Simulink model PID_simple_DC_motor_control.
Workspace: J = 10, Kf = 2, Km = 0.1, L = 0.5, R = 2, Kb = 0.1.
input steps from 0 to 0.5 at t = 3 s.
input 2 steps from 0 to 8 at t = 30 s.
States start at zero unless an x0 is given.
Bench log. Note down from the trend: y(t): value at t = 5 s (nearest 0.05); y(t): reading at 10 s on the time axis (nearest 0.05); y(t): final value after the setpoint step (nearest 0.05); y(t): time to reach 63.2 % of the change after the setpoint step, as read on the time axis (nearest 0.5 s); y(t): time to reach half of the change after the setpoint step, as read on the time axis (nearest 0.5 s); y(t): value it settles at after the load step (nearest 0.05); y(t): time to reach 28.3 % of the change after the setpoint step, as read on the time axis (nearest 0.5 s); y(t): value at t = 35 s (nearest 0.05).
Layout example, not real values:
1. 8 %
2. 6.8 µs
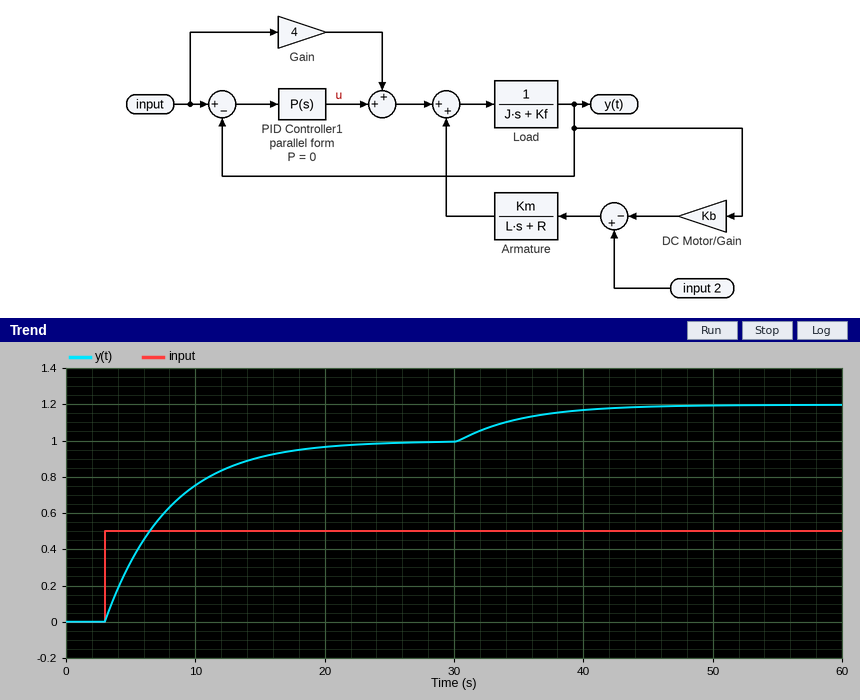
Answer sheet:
1. 0.35
2. 0.75
3. 1.00
4. 8.0 s
5. 6.5 s
6. 1.20
7. 4.5 s
8. 1.10
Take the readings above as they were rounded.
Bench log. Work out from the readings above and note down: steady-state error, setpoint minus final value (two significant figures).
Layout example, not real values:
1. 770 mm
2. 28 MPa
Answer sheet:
1. -0.50
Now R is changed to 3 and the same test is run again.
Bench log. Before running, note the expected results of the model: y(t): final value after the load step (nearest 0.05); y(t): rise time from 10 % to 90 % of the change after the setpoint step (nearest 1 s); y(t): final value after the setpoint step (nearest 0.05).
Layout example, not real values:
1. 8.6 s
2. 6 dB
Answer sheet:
1. 1.15
2. 11 s
3. 1.00
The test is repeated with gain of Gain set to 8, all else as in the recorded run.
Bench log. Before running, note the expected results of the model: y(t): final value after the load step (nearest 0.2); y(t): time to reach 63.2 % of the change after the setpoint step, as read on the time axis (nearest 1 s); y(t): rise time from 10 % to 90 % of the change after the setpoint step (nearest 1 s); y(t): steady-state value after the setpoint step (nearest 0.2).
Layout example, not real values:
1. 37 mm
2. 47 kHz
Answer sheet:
1. 2.2
2. 8 s
3. 11 s
4. 2.0
